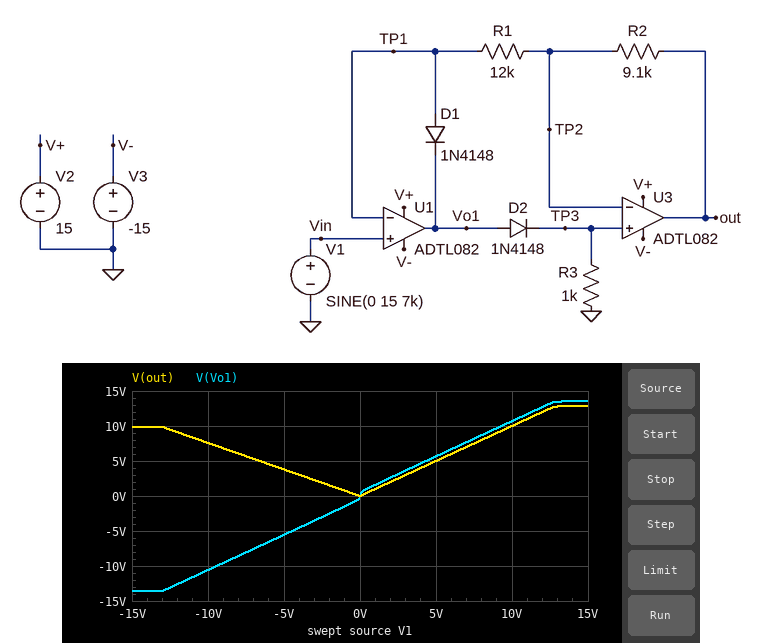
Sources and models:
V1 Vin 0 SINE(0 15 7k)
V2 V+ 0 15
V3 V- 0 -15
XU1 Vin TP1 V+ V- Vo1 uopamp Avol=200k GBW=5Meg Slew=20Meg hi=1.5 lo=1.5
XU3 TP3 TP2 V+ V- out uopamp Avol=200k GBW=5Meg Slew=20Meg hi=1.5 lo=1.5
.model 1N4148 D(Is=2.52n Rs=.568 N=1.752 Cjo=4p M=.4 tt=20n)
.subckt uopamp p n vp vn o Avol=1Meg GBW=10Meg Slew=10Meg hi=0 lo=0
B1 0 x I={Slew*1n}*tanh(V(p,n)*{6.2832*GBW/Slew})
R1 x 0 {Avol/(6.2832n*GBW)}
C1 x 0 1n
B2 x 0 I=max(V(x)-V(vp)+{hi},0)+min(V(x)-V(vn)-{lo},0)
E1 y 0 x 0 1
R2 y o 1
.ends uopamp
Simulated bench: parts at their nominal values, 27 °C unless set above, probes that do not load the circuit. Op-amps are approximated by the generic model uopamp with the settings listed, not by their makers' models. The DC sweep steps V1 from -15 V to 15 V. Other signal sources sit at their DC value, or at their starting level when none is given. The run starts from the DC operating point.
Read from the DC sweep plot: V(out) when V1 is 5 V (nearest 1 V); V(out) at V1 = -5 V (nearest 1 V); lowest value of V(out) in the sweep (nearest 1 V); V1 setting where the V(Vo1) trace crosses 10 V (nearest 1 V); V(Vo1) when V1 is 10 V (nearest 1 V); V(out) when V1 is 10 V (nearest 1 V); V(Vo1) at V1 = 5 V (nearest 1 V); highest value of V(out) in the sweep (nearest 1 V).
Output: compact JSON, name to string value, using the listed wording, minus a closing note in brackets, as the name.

{"V(out) when V1 is 5 V": "5 V", "V(out) at V1 = -5 V": "4 V", "lowest value of V(out) in the sweep": "0 V", "V1 setting where the V(Vo1) trace crosses 10 V": "9 V", "V(Vo1) when V1 is 10 V": "11 V", "V(out) when V1 is 10 V": "10 V", "V(Vo1) at V1 = 5 V": "6 V", "highest value of V(out) in the sweep": "13 V"}
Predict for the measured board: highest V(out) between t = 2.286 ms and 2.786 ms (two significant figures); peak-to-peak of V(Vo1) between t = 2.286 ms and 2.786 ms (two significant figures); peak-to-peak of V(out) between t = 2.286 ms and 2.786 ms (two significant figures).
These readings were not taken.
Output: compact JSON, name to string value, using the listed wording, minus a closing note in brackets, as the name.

{"highest V(out) between t = 2.286 ms and 2.786 ms": "13 V", "peak-to-peak of V(Vo1) between t = 2.286 ms and 2.786 ms": "27 V", "peak-to-peak of V(out) between t = 2.286 ms and 2.786 ms": "13 V"}
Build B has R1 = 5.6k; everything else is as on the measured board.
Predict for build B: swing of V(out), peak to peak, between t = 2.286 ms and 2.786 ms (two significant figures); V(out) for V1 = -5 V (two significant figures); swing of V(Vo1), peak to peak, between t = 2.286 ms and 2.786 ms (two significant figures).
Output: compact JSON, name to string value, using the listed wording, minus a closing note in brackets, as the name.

{"swing of V(out), peak to peak, between t = 2.286 ms and 2.786 ms": "14 V", "V(out) for V1 = -5 V": "8.1 V", "swing of V(Vo1), peak to peak, between t = 2.286 ms and 2.786 ms": "27 V"}
